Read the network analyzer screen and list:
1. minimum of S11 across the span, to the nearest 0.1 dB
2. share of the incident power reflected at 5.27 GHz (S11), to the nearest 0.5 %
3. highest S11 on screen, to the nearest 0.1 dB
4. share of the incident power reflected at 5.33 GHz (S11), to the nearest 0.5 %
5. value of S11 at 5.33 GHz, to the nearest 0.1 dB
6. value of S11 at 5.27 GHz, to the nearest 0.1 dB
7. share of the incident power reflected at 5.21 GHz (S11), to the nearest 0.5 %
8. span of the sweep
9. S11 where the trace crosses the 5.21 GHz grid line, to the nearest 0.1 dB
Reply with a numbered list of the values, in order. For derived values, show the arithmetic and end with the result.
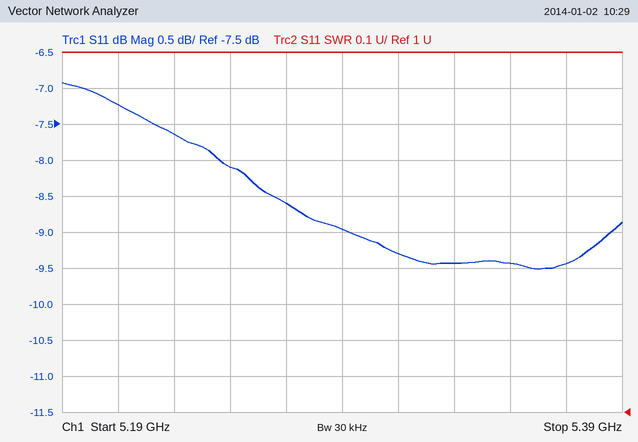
1. -9.5 dB
2. 10^(-8.6/10) ≈ 13.8 %, so 14.0 % to the nearest 0.5 %
3. -6.9 dB
4. 10^(-9.4/10) ≈ 11.5 %
5. -9.4 dB
6. -8.6 dB
7. 10^(-7.2/10) ≈ 19.1 %, so 19.0 % to the nearest 0.5 %
8. 200 MHz
9. -7.2 dB
